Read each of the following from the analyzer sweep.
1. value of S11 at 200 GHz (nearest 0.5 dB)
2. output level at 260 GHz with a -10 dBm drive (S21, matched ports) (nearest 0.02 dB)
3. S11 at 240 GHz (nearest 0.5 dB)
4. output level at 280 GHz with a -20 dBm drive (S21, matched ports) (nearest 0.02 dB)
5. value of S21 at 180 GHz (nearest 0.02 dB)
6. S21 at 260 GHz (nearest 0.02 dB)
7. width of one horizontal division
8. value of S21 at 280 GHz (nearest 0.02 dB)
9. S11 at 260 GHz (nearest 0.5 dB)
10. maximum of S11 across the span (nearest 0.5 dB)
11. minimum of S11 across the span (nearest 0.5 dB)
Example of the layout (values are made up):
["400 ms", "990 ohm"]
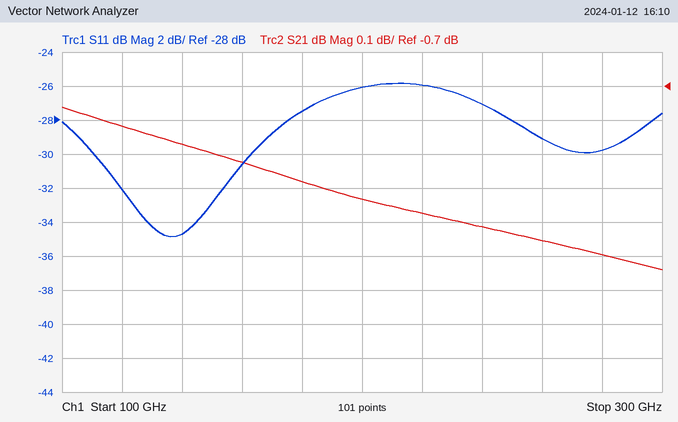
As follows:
["-26.0 dB", "-11.16 dBm", "-27.0 dB", "-21.20 dBm", "-0.98 dB", "-1.16 dB", "20 GHz", "-1.20 dB", "-29.0 dB", "-26.0 dB", "-35.0 dB"]
